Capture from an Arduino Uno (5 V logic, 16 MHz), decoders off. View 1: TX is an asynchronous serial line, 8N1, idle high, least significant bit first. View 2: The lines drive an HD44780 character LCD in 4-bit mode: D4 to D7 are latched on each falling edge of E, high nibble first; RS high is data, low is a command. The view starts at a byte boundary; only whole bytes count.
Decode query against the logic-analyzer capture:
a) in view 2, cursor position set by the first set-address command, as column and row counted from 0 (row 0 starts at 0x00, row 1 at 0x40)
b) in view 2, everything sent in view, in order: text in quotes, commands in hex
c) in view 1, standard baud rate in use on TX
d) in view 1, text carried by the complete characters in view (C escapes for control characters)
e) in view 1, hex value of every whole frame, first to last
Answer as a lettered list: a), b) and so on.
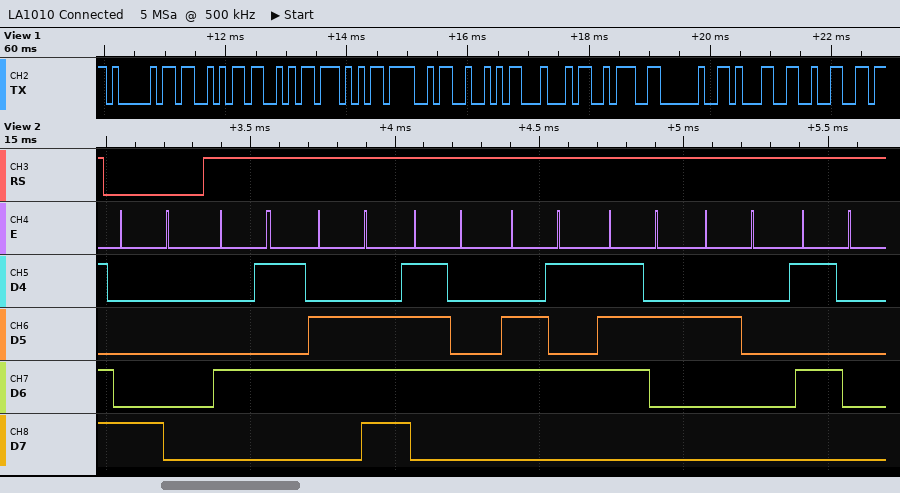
a) column 0, row 0
b) 0x80 "Enter P"
c) 9600 baud
d) "ASSWORD: 12"
e) 0x41 0x53 0x53 0x57 0x4F 0x52 0x44 0x3A 0x20 0x31 0x32
